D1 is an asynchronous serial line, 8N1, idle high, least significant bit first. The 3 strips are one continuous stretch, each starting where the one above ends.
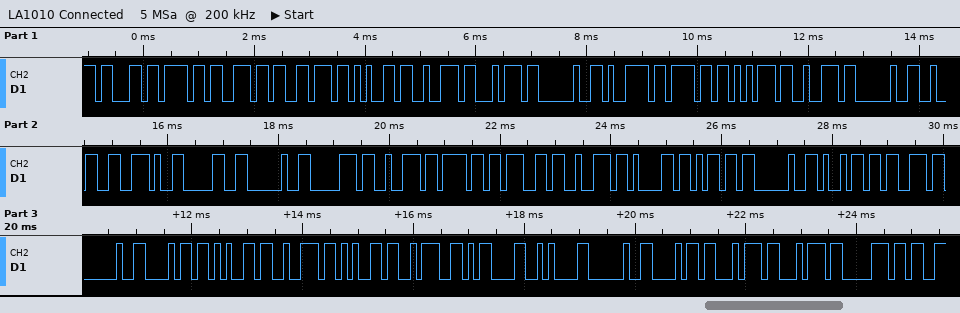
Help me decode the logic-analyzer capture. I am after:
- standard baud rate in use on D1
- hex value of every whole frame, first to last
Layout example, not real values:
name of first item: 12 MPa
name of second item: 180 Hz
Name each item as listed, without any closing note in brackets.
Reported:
standard baud rate in use on D1: 9600 baud
hex value of every whole frame, first to last: 63 6F 6E 76 65 72 74 20 79 6F 75 72 20 32 2E 30 20 70 72 6F 67 72 61 6D 20 69 73 20 68 65 72 65 3A 0D 0A 20 68 74 74 70
